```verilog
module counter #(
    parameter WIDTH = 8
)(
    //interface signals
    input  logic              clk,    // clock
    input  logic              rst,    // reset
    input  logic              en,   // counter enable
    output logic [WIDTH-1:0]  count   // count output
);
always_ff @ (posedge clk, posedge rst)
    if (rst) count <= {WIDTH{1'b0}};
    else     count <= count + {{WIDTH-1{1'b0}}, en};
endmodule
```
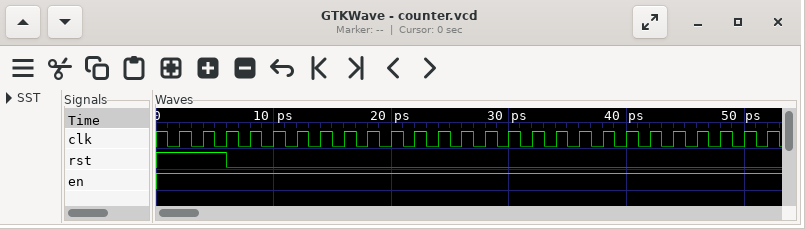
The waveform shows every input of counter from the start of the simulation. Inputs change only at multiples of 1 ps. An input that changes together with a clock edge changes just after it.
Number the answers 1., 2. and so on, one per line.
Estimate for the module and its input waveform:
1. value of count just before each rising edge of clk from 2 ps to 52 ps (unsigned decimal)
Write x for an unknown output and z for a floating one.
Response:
1. 0, 0, 0, 0, 1, 2, 3, 4, 5, 6, 7, 8, 9, 10, 11, 12, 13, 14, 15, 16, 17, 18, 19, 20, 21, 22
